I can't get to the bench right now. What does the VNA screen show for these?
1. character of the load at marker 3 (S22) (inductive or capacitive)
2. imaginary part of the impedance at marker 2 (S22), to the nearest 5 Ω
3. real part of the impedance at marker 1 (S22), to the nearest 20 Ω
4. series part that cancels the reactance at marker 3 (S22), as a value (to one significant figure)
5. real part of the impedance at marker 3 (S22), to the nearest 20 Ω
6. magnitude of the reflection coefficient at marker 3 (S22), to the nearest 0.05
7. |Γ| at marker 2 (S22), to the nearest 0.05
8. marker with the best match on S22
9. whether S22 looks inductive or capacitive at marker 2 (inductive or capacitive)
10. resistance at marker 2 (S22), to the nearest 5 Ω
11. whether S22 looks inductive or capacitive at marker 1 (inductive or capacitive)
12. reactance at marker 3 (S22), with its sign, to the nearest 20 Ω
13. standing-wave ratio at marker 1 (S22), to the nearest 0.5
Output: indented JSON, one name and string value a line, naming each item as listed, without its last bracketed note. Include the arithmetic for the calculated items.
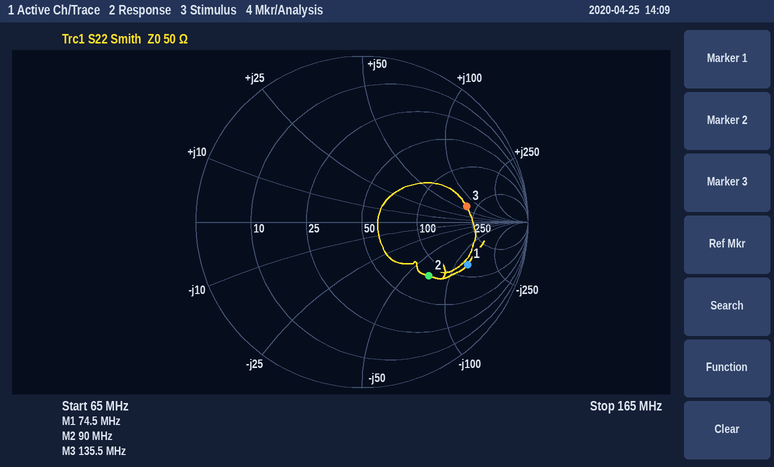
{
  "character of the load at marker 3 (S22)": "inductive",
  "imaginary part of the impedance at marker 2 (S22), to the nearest 5 Ω": "-70 Ω",
  "real part of the impedance at marker 1 (S22), to the nearest 20 Ω": "140 Ω",
  "series part that cancels the reactance at marker 3 (S22), as a value": "C = 1/(2π × 135.5 MHz × 60 Ω) ≈ 20 pF",
  "real part of the impedance at marker 3 (S22), to the nearest 20 Ω": "200 Ω",
  "magnitude of the reflection coefficient at marker 3 (S22), to the nearest 0.05": "0.65",
  "|Γ| at marker 2 (S22), to the nearest 0.05": "0.50",
  "marker with the best match on S22": "marker 2",
  "whether S22 looks inductive or capacitive at marker 2": "capacitive",
  "resistance at marker 2 (S22), to the nearest 5 Ω": "80 Ω",
  "whether S22 looks inductive or capacitive at marker 1": "capacitive",
  "reactance at marker 3 (S22), with its sign, to the nearest 20 Ω": "+60 Ω",
  "standing-wave ratio at marker 1 (S22), to the nearest 0.5": "5.5"
}
